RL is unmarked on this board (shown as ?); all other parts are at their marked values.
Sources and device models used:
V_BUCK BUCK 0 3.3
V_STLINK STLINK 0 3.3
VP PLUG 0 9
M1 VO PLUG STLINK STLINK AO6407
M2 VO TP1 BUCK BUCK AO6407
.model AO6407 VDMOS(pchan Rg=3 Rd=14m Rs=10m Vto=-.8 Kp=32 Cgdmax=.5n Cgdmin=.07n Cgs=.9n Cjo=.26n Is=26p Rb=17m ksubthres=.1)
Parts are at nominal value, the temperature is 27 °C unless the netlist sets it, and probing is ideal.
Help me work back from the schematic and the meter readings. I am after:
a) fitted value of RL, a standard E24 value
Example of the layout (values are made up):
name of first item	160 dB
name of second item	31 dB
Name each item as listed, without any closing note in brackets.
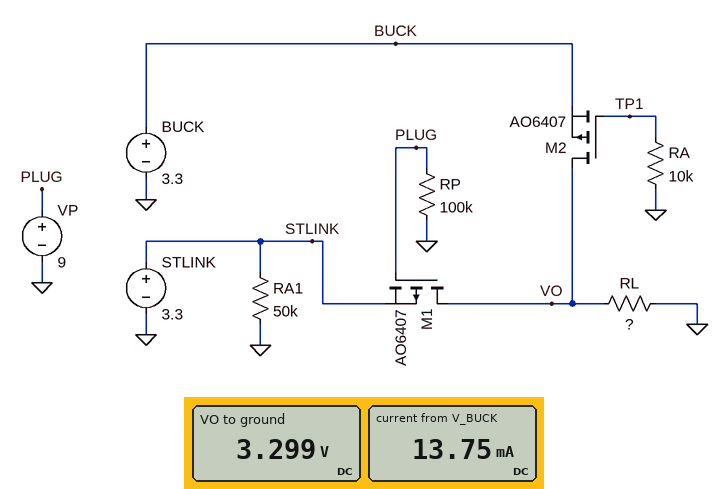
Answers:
fitted value of RL, a standard E24 value	240 Ω
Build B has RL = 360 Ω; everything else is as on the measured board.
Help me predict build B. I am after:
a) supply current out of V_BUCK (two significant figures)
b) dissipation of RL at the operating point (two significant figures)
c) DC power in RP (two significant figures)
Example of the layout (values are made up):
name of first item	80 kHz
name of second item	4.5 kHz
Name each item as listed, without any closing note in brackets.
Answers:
supply current out of V_BUCK	9.2 mA
dissipation of RL at the operating point	30 mW
DC power in RP	810 µW
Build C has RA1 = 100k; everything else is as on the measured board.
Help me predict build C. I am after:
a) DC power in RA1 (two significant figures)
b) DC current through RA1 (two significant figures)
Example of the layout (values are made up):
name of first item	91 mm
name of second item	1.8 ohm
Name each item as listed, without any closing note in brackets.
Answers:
DC power in RA1	110 µW
DC current through RA1	33 µA
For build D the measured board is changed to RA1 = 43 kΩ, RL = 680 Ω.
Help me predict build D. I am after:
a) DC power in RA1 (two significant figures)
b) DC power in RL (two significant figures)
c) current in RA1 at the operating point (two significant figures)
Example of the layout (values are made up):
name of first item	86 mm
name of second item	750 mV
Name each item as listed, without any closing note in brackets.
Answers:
DC power in RA1	250 µW
DC power in RL	16 mW
current in RA1 at the operating point	77 µA
